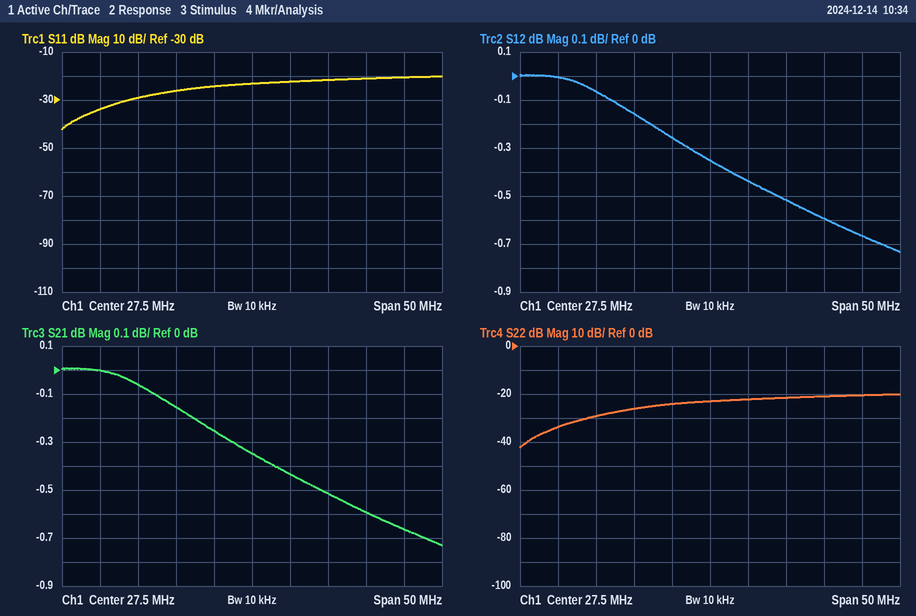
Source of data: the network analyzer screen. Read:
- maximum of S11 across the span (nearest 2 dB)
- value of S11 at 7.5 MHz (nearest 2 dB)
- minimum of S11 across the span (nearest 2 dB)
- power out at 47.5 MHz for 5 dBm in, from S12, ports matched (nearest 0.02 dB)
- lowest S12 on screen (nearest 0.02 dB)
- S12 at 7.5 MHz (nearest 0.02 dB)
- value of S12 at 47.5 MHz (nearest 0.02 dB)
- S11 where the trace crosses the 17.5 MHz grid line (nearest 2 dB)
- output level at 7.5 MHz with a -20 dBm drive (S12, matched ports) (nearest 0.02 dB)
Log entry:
-20 dB
-34 dB
-42 dB
4.34 dBm
-0.74 dB
0.00 dB
-0.66 dB
-26 dB
-20.00 dBm
